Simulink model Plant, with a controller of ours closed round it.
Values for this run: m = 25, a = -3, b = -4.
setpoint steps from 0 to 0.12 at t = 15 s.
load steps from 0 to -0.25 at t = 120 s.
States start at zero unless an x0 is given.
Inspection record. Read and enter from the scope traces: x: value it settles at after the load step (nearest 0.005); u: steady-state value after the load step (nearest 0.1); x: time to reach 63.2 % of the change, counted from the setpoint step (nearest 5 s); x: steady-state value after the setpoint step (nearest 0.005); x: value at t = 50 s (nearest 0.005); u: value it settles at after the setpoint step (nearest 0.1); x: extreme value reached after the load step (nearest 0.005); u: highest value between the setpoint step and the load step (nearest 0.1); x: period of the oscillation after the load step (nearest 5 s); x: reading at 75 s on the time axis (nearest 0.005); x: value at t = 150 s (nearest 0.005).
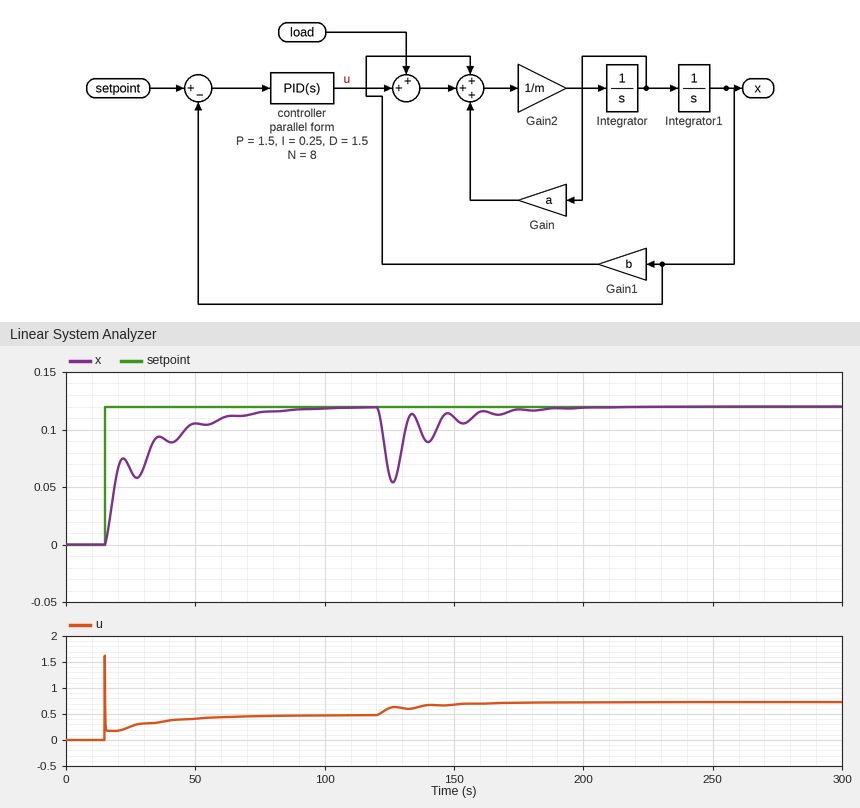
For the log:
0.120
0.7
15 s
0.120
0.105
0.5
0.055
1.6
15 s
0.115
0.110
